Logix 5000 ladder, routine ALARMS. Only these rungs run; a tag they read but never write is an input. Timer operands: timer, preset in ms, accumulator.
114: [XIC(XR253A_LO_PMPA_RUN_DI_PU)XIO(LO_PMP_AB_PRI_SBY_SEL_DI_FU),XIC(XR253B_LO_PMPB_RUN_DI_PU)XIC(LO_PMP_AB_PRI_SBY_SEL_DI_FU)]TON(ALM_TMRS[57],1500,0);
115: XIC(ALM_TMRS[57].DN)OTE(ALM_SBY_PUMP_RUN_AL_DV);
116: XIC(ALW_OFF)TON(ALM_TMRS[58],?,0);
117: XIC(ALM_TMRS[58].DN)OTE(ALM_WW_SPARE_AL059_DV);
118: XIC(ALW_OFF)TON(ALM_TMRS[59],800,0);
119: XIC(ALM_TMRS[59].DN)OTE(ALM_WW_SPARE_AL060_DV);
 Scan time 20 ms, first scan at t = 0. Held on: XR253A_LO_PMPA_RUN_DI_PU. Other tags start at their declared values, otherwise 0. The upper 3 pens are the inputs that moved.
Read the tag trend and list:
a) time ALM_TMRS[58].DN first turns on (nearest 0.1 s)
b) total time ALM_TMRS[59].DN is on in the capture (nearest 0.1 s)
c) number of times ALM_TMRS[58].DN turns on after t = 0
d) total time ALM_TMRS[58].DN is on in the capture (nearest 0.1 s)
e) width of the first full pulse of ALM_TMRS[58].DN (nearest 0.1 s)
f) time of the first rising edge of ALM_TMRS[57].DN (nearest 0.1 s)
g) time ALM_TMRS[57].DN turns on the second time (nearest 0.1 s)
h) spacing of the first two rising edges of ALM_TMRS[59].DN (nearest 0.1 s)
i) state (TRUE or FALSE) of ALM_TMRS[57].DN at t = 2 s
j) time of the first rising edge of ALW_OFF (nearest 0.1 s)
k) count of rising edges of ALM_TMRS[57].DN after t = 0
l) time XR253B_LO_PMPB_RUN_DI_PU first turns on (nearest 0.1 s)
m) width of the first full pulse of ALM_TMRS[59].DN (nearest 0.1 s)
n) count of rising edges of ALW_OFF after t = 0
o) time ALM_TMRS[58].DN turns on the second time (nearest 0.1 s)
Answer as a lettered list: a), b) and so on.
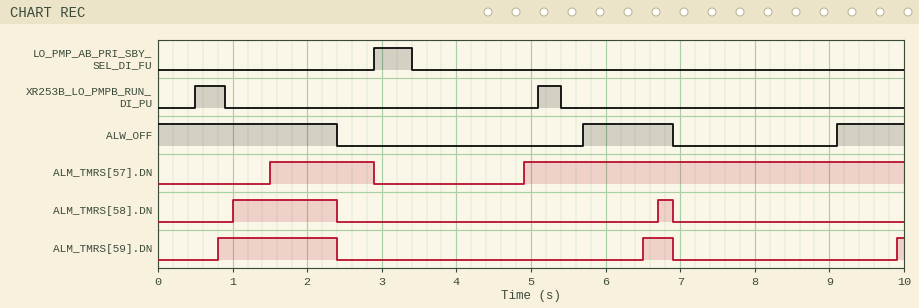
a) 1.0 s
b) 2.1 s
c) 2
d) 1.6 s
e) 1.4 s
f) 1.5 s
g) 4.9 s
h) 5.7 s
i) TRUE
j) 5.7 s
k) 2
l) 0.5 s
m) 1.6 s
n) 2
o) 6.7 s
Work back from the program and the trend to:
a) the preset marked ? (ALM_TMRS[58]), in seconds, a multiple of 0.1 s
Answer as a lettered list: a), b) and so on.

a) 1.0 s
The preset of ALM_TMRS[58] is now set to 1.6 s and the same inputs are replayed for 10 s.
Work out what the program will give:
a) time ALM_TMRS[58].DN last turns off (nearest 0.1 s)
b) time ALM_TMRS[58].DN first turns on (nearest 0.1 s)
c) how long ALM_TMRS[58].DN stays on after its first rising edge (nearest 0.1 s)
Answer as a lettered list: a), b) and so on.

a) 2.4 s
b) 1.6 s
c) 0.8 s
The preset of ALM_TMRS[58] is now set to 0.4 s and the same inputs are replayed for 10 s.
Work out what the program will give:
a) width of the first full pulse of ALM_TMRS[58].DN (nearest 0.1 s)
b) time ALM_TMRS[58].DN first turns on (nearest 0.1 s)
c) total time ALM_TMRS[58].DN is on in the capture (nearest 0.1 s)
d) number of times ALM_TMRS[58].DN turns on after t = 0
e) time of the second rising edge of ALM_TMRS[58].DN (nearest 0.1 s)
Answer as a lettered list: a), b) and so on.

a) 2.0 s
b) 0.4 s
c) 3.3 s
d) 3
e) 6.1 s
